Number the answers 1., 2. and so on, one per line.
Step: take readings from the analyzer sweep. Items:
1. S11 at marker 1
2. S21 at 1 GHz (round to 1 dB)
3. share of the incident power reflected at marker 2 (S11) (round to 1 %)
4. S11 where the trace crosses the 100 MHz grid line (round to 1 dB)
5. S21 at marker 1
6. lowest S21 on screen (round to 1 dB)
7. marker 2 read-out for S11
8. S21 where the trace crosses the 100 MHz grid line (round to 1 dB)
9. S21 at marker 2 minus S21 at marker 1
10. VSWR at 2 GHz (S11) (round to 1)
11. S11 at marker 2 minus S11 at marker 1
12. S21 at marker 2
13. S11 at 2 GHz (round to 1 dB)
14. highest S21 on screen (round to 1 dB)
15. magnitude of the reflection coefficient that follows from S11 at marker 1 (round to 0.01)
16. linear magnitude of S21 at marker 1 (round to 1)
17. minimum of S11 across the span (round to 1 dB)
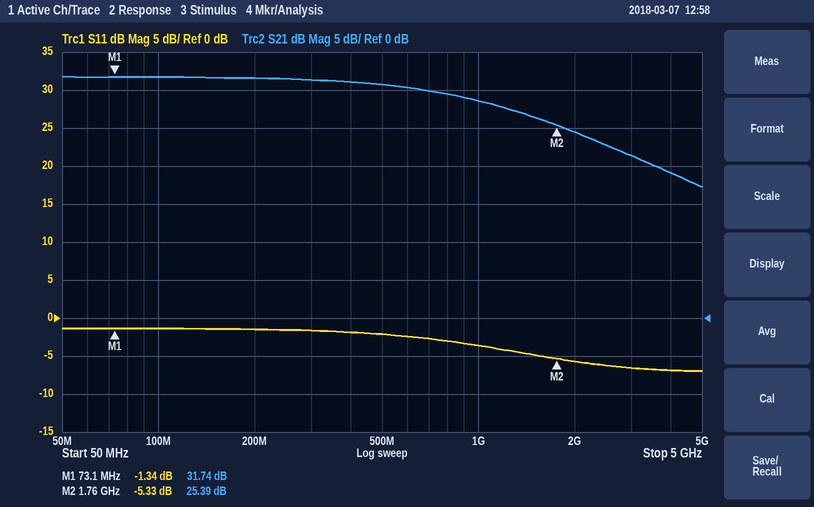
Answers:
1. -1.34 dB
2. 29 dB
3. 29 %
4. -1 dB
5. 31.74 dB
6. 17 dB
7. -5.33 dB
8. 32 dB
9. -6.35 dB
10. 3
11. -3.99 dB
12. 25.39 dB
13. -6 dB
14. 32 dB
15. 0.86
16. 39
17. -7 dB
